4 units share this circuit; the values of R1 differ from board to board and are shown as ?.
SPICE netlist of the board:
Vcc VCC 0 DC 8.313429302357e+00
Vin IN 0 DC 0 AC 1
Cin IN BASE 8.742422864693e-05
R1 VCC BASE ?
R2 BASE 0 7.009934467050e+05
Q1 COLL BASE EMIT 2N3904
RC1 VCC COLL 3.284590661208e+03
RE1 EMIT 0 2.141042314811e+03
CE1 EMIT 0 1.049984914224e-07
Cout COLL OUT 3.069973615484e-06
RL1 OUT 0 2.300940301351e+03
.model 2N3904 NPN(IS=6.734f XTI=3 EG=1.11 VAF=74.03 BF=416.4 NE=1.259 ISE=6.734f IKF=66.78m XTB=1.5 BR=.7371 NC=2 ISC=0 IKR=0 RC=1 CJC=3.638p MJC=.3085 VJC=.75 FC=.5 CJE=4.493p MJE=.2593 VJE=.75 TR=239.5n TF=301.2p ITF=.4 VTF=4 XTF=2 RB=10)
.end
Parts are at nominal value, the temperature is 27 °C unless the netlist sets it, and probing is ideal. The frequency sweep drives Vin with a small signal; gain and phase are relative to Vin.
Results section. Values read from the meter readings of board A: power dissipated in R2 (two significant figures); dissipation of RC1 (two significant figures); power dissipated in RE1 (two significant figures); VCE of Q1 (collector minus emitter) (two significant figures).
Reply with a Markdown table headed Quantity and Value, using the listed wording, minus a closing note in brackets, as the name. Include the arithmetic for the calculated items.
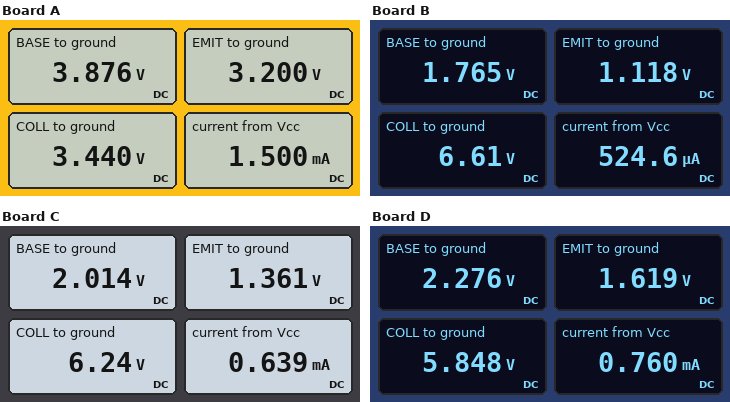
| Quantity | Value |
|---|---|
| power dissipated in R2 | (3.876 V)^2 / 701 kΩ = 21 µW |
| dissipation of RC1 | (8.313 V - 3.44 V)^2 / 3.285 kΩ = 7.2 mW |
| power dissipated in RE1 | (3.2 V)^2 / 2.141 kΩ = 4.8 mW |
| VCE of Q1 (collector minus emitter) | 3.44 V - 3.2 V = 240 mV |
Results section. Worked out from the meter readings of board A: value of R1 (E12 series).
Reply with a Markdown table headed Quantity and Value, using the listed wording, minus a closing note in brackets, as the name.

| Quantity | Value |
|---|---|
| value of R1 | 270 kΩ |
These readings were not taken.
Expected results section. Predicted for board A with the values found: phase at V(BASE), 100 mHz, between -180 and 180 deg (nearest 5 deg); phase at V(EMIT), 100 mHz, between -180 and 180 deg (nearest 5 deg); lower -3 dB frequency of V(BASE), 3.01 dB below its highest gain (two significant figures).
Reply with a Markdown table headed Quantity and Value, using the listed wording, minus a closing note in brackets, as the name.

| Quantity | Value |
|---|---|
| phase at V(BASE), 100 mHz, between -180 and 180 deg | 25 deg |
| phase at V(EMIT), 100 mHz, between -180 and 180 deg | 25 deg |
| lower -3 dB frequency of V(BASE), 3.01 dB below its highest gain | 50 mHz |
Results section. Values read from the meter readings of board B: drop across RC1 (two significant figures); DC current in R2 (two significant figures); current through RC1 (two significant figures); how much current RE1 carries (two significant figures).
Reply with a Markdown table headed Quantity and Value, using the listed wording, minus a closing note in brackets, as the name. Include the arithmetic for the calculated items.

| Quantity | Value |
|---|---|
| drop across RC1 | 8.313 V - 6.61 V = 1.7 V |
| DC current in R2 | (1.765 V) / 701 kΩ = 2.5 µA |
| current through RC1 | (8.313 V - 6.61 V) / 3.285 kΩ = 520 µA |
| how much current RE1 carries | (1.118 V) / 2.141 kΩ = 520 µA |
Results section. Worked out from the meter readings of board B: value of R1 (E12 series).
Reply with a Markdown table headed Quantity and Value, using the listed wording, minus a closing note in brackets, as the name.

| Quantity | Value |
|---|---|
| value of R1 | 1 MΩ |
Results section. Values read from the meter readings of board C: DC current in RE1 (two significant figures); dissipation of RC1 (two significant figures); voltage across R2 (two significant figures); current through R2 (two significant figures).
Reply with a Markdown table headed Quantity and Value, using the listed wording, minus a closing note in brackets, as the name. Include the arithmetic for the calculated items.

| Quantity | Value |
|---|---|
| DC current in RE1 | (1.361 V) / 2.141 kΩ = 640 µA |
| dissipation of RC1 | (8.313 V - 6.24 V)^2 / 3.285 kΩ = 1.3 mW |
| voltage across R2 | 2.014 V = 2.0 V |
| current through R2 | (2.014 V) / 701 kΩ = 2.9 µA |
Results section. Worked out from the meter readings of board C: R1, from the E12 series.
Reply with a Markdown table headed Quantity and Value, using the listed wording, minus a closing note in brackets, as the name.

| Quantity | Value |
|---|---|
| R1, from the E12 series | 820 kΩ |
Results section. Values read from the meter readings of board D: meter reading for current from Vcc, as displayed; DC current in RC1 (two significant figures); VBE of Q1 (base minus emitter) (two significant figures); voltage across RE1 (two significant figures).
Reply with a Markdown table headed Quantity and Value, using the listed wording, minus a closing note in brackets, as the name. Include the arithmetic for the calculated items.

| Quantity | Value |
|---|---|
| meter reading for current from Vcc, as displayed | 0.760 mA |
| DC current in RC1 | (8.313 V - 5.848 V) / 3.285 kΩ = 750 µA |
| VBE of Q1 (base minus emitter) | 2.276 V - 1.619 V = 660 mV |
| voltage across RE1 | 1.619 V = 1.6 V |
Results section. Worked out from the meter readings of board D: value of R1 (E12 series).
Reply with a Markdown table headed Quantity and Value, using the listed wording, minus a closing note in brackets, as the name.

| Quantity | Value |
|---|---|
| value of R1 | 680 kΩ |
